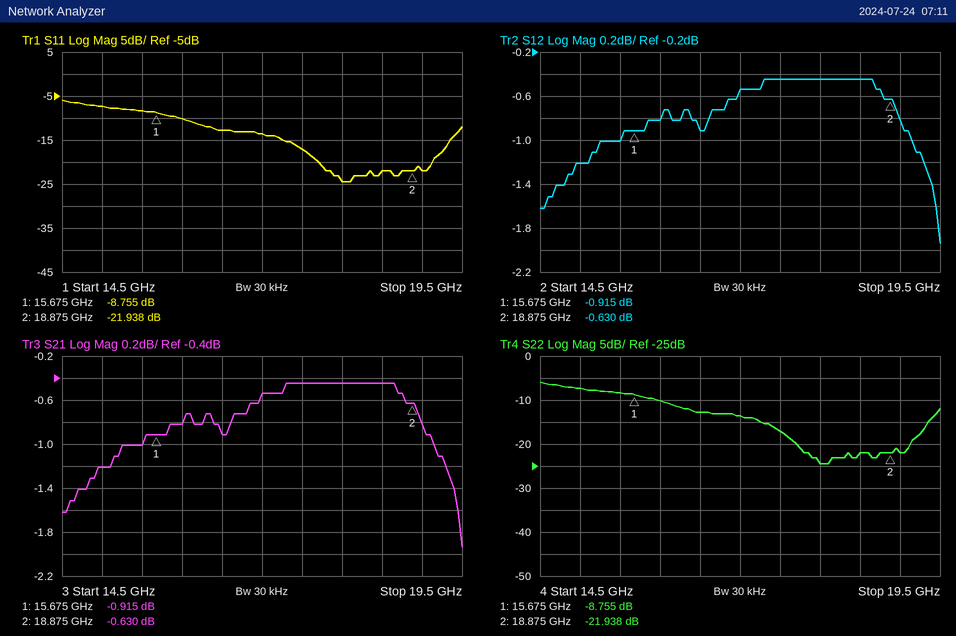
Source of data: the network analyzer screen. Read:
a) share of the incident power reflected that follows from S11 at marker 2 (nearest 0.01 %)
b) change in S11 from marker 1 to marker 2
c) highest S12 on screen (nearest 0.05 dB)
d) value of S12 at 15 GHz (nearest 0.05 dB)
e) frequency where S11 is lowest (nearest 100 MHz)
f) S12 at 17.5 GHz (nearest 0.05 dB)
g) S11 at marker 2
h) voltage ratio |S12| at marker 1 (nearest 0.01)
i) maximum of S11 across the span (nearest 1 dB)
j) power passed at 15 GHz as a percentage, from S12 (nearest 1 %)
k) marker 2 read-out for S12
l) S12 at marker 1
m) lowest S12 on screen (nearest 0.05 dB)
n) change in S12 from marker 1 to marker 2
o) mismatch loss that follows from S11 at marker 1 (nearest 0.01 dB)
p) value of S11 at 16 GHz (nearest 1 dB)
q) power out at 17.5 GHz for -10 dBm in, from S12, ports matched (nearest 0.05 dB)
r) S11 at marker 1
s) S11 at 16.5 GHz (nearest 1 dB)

0.64 %
-13.183 dB
-0.45 dB
-1.20 dB
18.0 GHz
-0.45 dB
-21.938 dB
0.90
-6 dB
76 %
-0.630 dB
-0.915 dB
-1.95 dB
0.285 dB
0.62 dB
-10 dB
-10.45 dBm
-8.755 dB
-13 dB
